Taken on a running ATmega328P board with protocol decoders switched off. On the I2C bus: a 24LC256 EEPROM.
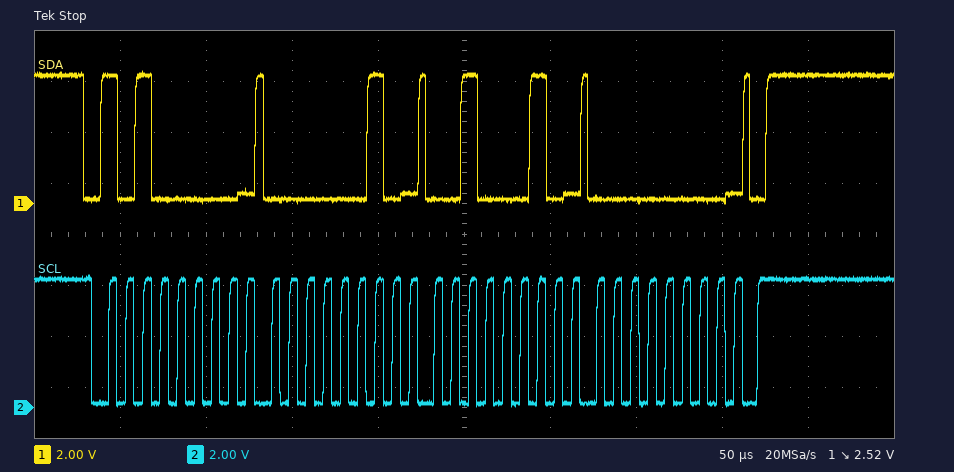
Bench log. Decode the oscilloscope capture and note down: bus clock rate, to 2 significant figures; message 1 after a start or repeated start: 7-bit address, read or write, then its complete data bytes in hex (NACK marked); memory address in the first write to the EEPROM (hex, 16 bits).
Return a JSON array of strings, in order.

["100 kHz", "0x50 write: 02 22 00", "0x0222"]
